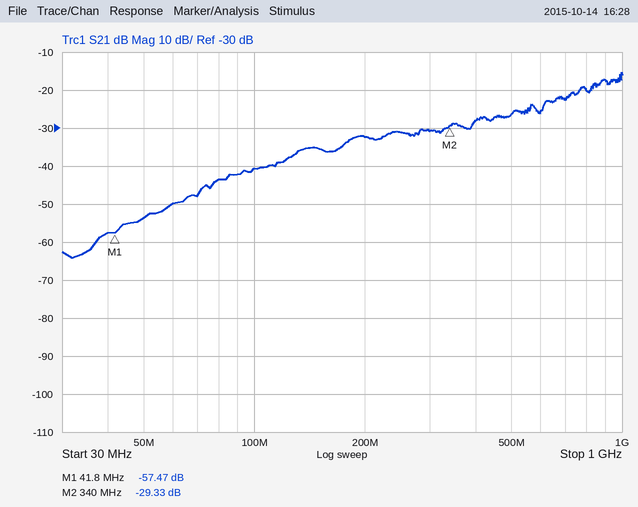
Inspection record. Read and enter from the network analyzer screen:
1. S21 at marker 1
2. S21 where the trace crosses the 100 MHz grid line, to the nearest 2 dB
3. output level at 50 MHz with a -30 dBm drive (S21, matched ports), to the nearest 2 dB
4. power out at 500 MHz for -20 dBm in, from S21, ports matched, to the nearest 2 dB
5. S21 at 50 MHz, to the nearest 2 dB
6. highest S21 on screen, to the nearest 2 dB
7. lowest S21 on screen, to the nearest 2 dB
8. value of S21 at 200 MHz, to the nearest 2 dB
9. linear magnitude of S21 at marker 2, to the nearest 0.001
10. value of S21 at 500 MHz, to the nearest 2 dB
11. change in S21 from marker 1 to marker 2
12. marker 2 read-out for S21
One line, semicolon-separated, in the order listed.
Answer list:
-57.47 dB; -40 dB; -84 dBm; -46 dBm; -54 dB; -16 dB; -64 dB; -32 dB; 0.034; -26 dB; 28.14 dB; -29.33 dB
